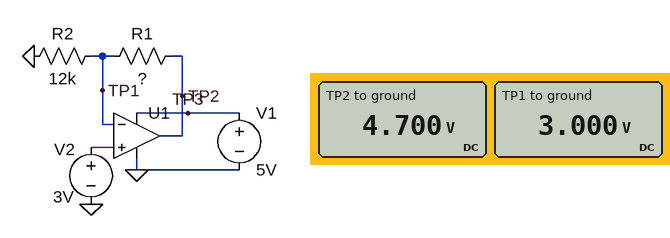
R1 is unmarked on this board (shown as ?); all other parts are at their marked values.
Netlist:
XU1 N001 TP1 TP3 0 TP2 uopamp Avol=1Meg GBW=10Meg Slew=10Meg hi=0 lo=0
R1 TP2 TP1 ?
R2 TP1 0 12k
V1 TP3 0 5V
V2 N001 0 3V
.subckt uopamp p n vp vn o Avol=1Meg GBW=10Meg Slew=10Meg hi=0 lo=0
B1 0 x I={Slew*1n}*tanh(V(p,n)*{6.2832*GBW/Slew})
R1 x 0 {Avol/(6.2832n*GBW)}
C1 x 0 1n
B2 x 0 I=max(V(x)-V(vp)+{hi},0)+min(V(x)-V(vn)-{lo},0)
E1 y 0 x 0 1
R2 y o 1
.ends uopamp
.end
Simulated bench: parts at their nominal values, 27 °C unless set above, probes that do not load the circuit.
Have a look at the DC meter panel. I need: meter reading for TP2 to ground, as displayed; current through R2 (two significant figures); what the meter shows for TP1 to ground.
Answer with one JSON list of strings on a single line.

["4.700 V", "250 µA", "3.000 V"]
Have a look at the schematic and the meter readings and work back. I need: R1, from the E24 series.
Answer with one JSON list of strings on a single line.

["6.8 kΩ"]
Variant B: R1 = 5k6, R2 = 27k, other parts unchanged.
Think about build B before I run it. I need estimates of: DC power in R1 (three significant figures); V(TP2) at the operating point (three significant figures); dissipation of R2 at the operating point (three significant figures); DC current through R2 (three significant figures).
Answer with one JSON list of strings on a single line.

["69.1 µW", "3.62 V", "333 µW", "111 µA"]
